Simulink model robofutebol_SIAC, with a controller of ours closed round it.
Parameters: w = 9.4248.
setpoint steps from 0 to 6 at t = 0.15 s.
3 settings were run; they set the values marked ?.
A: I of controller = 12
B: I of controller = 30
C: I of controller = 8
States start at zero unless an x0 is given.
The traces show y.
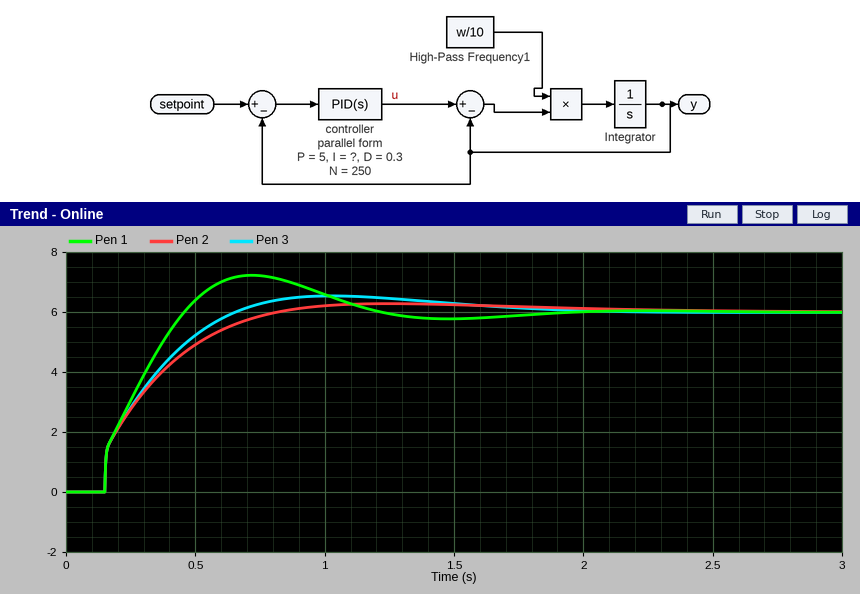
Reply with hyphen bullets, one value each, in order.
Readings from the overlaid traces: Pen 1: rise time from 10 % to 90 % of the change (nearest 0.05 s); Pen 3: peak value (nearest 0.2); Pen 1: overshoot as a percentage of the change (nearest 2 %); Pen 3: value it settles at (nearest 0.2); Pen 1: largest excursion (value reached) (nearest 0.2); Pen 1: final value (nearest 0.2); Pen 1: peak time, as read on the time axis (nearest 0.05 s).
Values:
- 0.25 s
- 6.6
- 20 %
- 6.0
- 7.2
- 6.0
- 0.70 s
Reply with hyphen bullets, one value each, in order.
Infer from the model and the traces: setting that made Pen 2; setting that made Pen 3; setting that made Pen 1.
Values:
- C
- A
- B
